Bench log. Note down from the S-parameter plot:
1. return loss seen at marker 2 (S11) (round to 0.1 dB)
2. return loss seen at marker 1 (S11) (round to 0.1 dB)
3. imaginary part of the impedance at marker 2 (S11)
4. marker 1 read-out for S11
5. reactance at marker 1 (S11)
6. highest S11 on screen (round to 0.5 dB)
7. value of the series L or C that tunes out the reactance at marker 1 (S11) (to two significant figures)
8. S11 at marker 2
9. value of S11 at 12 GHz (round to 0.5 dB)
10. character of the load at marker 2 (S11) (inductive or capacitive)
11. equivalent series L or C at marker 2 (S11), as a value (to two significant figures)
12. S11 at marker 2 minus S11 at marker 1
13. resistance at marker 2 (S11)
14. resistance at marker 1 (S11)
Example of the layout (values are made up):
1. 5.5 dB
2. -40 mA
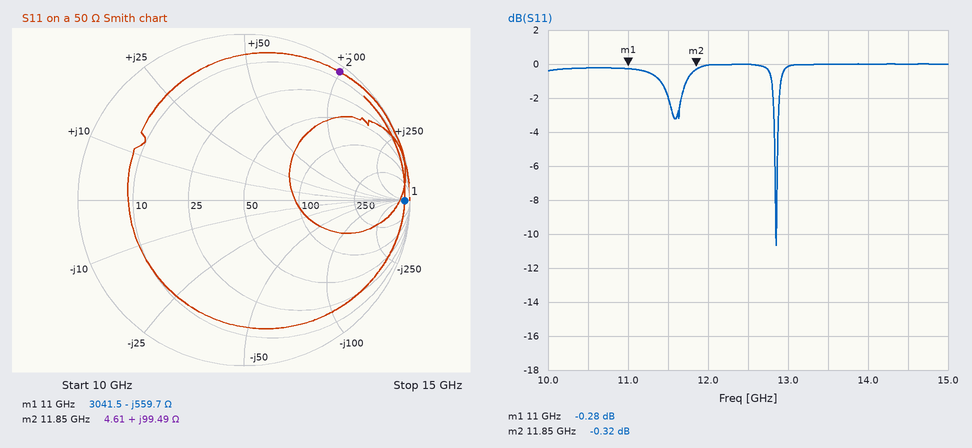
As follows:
1. 0.3 dB
2. 0.3 dB
3. +99.49 Ω
4. -0.28 dB
5. -559.7 Ω
6. 0.0 dB
7. 8.1 nH
8. -0.32 dB
9. 0.0 dB
10. inductive
11. 1.3 nH
12. -0.04 dB
13. 4.61 Ω
14. 3041.5 Ω
